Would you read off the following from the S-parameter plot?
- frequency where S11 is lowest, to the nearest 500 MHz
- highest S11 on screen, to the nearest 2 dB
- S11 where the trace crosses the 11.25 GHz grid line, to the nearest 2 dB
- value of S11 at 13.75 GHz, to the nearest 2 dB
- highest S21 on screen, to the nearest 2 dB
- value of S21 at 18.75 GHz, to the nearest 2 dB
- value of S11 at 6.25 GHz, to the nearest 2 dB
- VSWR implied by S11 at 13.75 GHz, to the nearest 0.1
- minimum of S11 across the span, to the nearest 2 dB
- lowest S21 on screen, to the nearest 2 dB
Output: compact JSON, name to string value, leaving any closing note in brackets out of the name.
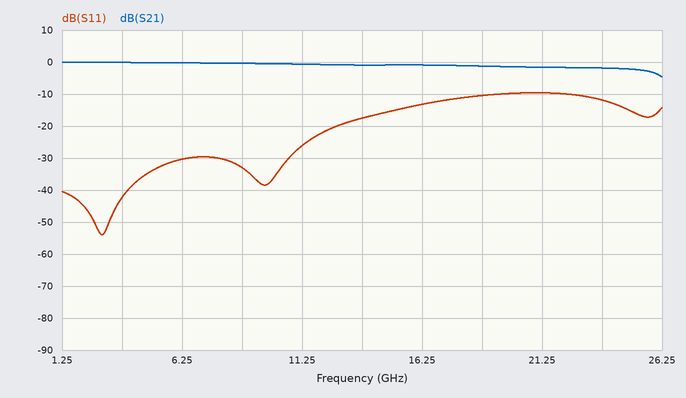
{"frequency where S11 is lowest, to the nearest 500 MHz": "3.0 GHz", "highest S11 on screen, to the nearest 2 dB": "-10 dB", "S11 where the trace crosses the 11.25 GHz grid line, to the nearest 2 dB": "-26 dB", "value of S11 at 13.75 GHz, to the nearest 2 dB": "-18 dB", "highest S21 on screen, to the nearest 2 dB": "0 dB", "value of S21 at 18.75 GHz, to the nearest 2 dB": "-2 dB", "value of S11 at 6.25 GHz, to the nearest 2 dB": "-30 dB", "VSWR implied by S11 at 13.75 GHz, to the nearest 0.1": "1.3", "minimum of S11 across the span, to the nearest 2 dB": "-54 dB", "lowest S21 on screen, to the nearest 2 dB": "-4 dB"}
